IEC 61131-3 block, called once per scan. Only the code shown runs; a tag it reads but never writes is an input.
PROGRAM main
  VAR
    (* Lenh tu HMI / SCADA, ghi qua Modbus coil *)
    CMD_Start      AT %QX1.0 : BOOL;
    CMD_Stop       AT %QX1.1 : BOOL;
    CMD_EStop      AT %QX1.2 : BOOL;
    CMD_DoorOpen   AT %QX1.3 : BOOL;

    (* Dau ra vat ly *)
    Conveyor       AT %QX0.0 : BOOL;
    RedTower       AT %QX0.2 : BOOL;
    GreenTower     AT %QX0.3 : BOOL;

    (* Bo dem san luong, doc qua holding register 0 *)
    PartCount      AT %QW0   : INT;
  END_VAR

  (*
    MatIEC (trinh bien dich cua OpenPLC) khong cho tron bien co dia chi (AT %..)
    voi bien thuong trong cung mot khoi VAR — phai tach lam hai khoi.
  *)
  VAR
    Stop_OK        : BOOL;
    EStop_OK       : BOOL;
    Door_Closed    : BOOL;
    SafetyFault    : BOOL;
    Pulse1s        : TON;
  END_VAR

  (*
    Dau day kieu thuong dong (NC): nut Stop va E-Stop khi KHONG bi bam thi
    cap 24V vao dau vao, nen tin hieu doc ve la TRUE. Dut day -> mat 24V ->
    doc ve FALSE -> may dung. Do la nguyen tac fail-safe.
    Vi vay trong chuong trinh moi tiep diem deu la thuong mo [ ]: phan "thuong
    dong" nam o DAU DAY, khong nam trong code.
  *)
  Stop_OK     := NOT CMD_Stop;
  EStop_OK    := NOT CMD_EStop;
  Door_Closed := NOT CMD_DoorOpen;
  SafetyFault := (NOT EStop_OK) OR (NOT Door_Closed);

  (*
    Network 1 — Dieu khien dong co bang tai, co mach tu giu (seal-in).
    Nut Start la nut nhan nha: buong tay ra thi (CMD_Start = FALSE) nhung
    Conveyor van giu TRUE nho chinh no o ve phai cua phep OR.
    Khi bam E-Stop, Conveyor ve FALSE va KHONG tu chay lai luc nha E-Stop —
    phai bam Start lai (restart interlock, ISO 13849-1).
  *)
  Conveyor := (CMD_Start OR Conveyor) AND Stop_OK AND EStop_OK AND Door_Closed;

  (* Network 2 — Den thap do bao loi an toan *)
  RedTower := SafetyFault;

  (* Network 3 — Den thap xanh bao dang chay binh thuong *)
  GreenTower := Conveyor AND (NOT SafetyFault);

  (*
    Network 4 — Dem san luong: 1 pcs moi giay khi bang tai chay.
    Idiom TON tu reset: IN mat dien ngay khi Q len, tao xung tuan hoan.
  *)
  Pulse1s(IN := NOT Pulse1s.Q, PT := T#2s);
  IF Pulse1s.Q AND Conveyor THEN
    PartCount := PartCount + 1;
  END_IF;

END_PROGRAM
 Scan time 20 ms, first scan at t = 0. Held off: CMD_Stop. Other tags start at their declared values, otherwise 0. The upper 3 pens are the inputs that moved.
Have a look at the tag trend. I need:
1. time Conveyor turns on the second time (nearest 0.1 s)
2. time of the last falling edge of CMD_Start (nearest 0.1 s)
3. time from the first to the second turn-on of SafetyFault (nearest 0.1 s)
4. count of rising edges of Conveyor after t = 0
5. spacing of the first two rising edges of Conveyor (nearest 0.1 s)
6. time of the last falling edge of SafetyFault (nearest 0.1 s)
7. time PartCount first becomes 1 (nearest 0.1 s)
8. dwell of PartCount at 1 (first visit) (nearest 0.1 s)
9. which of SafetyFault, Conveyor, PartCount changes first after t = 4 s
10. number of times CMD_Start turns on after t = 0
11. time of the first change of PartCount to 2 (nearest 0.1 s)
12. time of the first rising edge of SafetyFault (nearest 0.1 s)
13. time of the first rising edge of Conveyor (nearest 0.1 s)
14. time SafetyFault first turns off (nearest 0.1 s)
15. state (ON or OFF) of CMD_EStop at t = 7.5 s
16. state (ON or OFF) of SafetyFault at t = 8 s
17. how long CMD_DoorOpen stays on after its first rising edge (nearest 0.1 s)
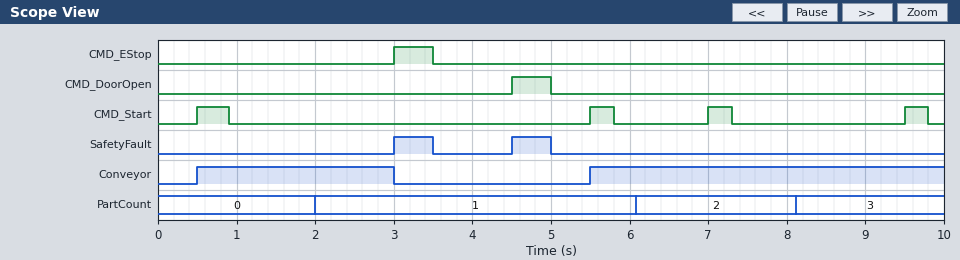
5.5 s
9.8 s
1.5 s
2
5.0 s
5.0 s
2.0 s
4.1 s
SafetyFault
4
6.1 s
3.0 s
0.5 s
3.5 s
OFF
OFF
0.5 s
